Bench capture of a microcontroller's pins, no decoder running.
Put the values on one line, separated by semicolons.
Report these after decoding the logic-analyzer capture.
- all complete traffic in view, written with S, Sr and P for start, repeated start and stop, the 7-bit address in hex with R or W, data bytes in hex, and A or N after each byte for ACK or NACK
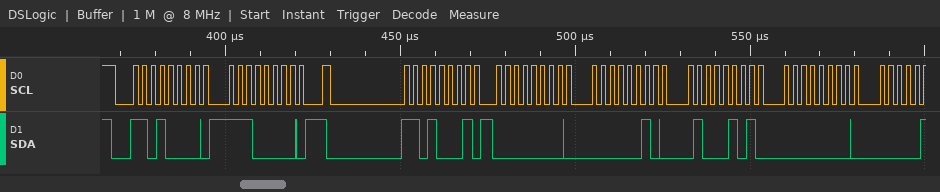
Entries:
S 68W A E0 A Sr 68R A 00 A 02 A 45 A 00 A
